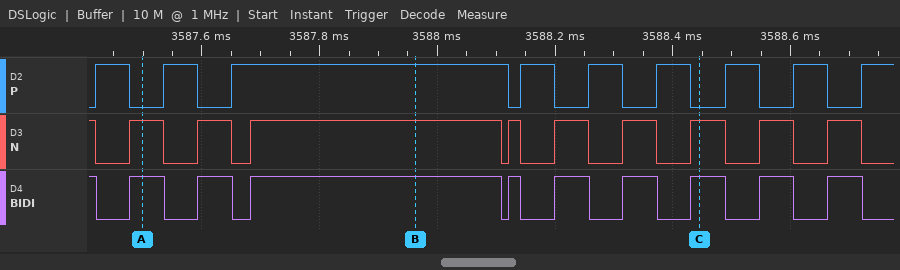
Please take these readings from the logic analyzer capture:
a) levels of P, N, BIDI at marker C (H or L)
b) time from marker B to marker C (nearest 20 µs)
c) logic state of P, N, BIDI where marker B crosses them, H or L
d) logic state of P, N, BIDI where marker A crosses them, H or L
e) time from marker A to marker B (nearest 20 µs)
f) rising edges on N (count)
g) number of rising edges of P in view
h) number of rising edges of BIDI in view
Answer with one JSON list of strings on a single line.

["P=L, N=H, BIDI=H", "480 µs", "P=H, N=H, BIDI=H", "P=L, N=H, BIDI=H", "460 µs", "9", "9", "9"]
